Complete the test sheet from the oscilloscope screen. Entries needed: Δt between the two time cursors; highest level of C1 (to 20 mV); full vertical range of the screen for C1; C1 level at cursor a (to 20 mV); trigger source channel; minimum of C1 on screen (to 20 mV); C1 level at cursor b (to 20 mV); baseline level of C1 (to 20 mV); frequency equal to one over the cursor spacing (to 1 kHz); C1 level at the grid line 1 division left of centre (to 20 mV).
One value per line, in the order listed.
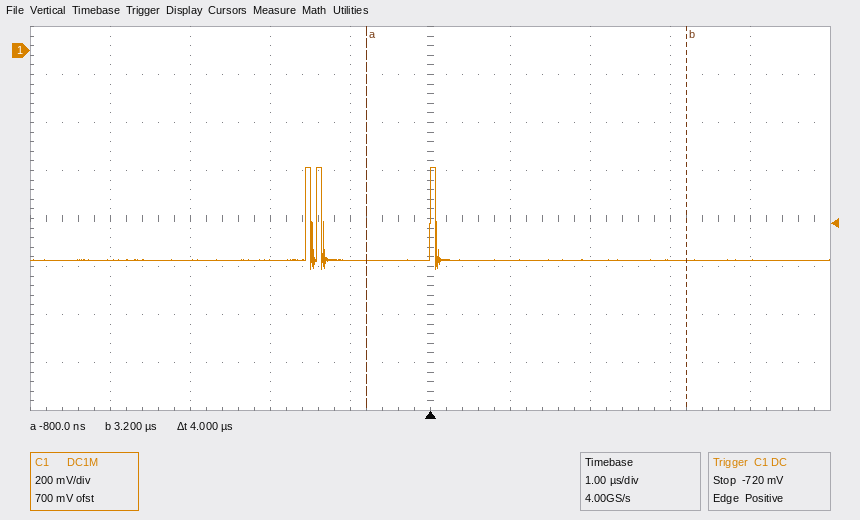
4 µs
-480 mV
1.6 V
-880 mV
C1
-920 mV
-880 mV
-880 mV
250 kHz
-880 mV
